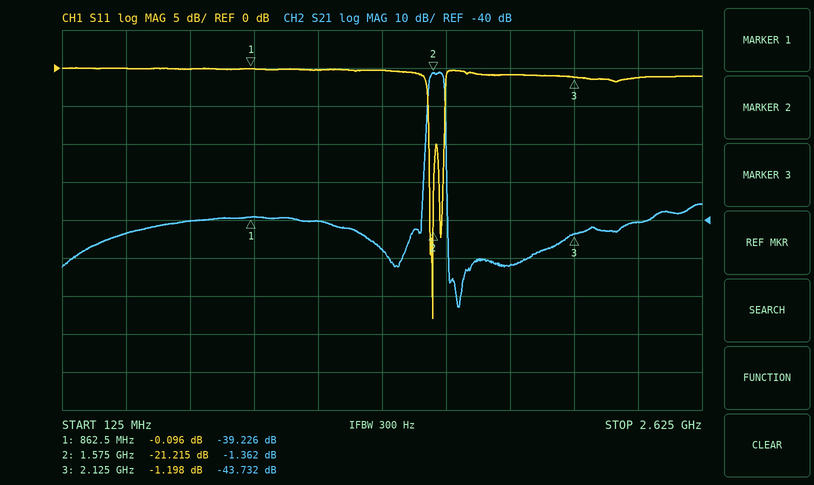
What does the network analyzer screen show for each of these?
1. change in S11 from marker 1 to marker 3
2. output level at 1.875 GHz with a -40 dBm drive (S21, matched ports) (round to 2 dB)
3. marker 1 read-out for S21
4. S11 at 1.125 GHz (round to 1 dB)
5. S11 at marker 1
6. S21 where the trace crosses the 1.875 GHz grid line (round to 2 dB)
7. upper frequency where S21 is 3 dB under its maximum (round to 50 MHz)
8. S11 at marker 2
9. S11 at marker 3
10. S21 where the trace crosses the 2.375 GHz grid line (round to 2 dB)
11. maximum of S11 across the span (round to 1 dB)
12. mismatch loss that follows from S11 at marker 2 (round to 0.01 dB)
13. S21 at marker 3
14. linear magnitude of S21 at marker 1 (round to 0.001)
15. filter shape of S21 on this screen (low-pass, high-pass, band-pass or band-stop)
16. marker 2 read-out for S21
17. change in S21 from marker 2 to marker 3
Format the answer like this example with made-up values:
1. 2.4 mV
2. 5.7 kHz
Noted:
1. -1.102 dB
2. -92 dBm
3. -39.226 dB
4. 0 dB
5. -0.096 dB
6. -52 dB
7. 1.60 GHz
8. -21.215 dB
9. -1.198 dB
10. -40 dB
11. 0 dB
12. 0.03 dB
13. -43.732 dB
14. 0.011
15. band-pass
16. -1.362 dB
17. -42.370 dB
